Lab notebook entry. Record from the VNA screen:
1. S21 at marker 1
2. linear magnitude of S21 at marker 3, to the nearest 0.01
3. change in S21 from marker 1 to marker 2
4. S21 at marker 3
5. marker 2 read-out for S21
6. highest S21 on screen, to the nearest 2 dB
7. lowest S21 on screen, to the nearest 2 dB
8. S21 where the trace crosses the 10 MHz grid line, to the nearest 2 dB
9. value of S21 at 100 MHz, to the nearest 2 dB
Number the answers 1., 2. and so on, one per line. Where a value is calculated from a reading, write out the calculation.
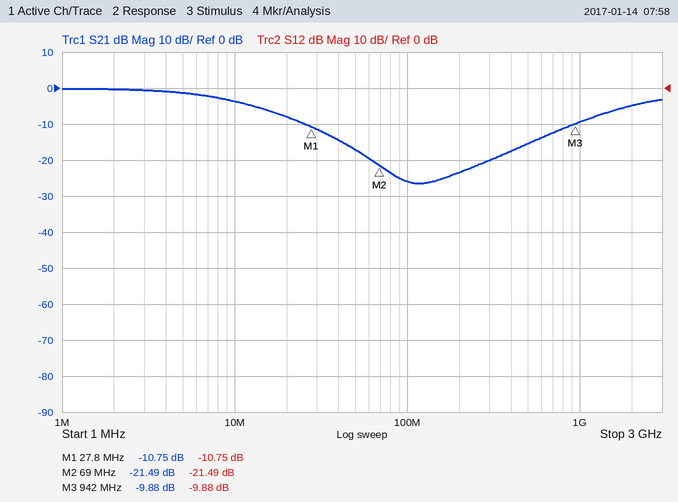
1. -10.75 dB
2. 10^(-9.88/20) ≈ 0.32
3. -21.49 − (-10.75) = -10.74 dB
4. -9.88 dB
5. -21.49 dB
6. 0 dB
7. -26 dB
8. -4 dB
9. -26 dB
